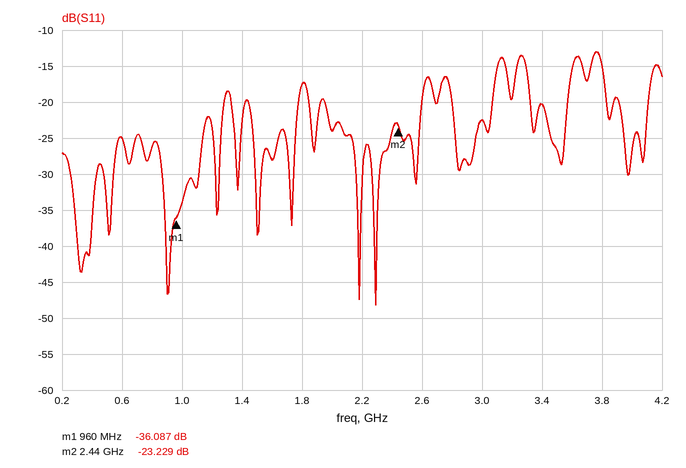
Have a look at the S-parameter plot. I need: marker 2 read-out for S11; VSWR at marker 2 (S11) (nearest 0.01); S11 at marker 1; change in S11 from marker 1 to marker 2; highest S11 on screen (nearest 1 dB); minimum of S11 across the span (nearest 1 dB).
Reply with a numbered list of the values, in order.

1. -23.229 dB
2. 1.15
3. -36.087 dB
4. 12.858 dB
5. -13 dB
6. -48 dB
